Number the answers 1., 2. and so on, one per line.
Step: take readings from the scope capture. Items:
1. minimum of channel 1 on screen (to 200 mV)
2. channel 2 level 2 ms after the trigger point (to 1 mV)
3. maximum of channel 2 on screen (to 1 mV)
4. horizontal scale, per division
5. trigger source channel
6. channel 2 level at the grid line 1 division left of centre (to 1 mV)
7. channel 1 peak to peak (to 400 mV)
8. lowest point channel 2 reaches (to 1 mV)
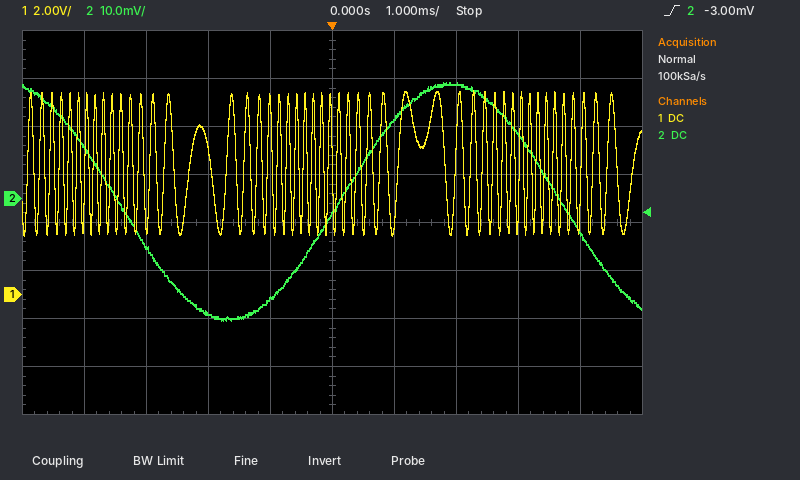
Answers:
1. 2.4 V
2. 24 mV
3. 24 mV
4. 1 ms
5. channel 2
6. -21 mV
7. 6.0 V
8. -25 mV
